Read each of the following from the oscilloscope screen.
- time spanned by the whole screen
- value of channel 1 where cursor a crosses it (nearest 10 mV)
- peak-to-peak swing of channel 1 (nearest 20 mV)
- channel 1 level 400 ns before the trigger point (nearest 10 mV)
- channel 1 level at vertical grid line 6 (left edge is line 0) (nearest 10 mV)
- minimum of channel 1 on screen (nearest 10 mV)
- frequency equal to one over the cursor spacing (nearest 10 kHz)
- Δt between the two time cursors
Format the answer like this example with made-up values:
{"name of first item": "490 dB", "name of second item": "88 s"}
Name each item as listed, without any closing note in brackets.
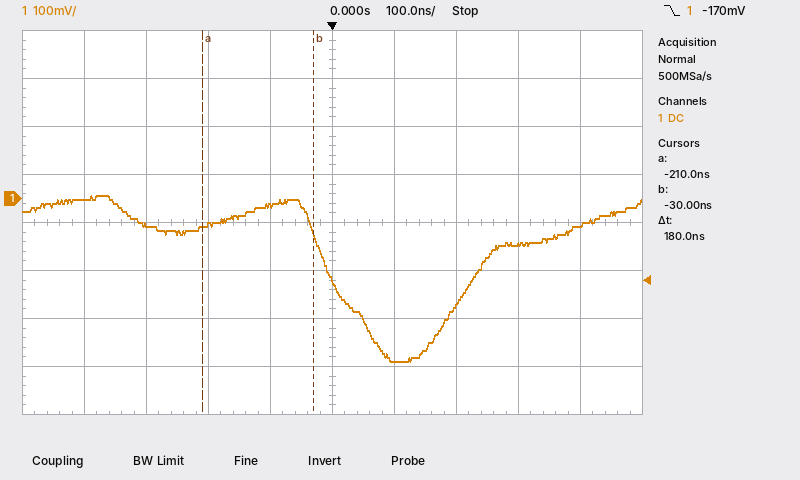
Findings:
{"time spanned by the whole screen": "1 µs", "value of channel 1 where cursor a crosses it": "-60 mV", "peak-to-peak swing of channel 1": "340 mV", "channel 1 level 400 ns before the trigger point": "0 mV", "channel 1 level at vertical grid line 6 (left edge is line 0)": "-340 mV", "minimum of channel 1 on screen": "-340 mV", "frequency equal to one over the cursor spacing": "5.56 MHz", "Δt between the two time cursors": "180 ns"}
